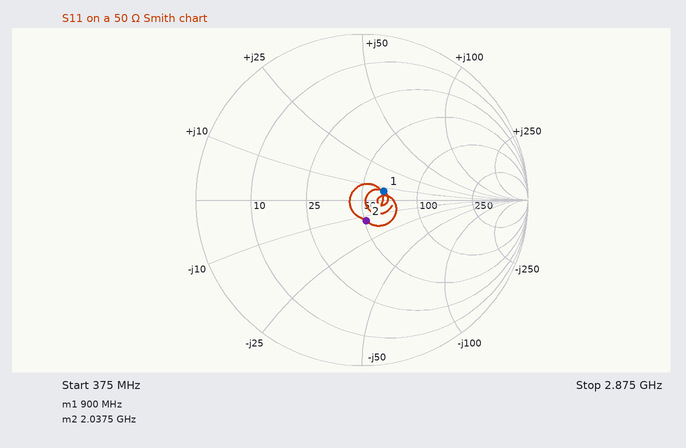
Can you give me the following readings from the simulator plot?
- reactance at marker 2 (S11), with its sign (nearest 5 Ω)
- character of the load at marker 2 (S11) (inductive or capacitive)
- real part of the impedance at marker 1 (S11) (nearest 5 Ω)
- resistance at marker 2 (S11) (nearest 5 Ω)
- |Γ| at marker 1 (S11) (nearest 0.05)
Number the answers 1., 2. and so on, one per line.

1. -15 Ω
2. capacitive
3. 65 Ω
4. 50 Ω
5. 0.15
